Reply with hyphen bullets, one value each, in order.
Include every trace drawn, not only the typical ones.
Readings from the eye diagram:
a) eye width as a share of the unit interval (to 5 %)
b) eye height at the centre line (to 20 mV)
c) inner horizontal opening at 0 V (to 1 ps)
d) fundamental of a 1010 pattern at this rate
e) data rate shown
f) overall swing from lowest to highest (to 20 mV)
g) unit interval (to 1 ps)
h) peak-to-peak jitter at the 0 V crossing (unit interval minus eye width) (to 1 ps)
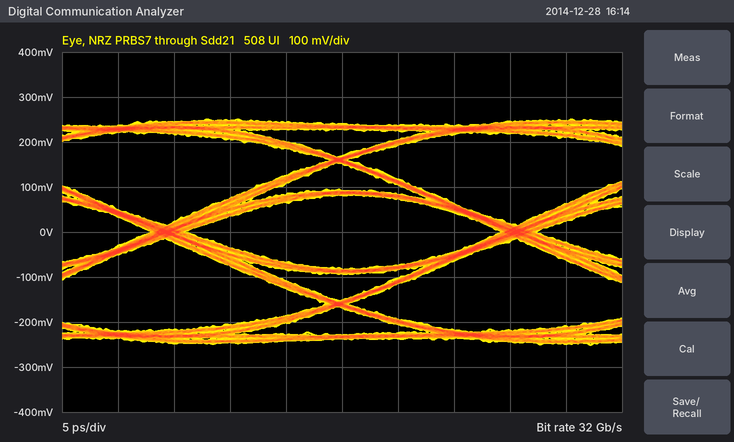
- 90 %
- 160 mV
- 28 ps
- 16 GHz
- 32 Gb/s
- 500 mV
- 31 ps
- 3 ps
